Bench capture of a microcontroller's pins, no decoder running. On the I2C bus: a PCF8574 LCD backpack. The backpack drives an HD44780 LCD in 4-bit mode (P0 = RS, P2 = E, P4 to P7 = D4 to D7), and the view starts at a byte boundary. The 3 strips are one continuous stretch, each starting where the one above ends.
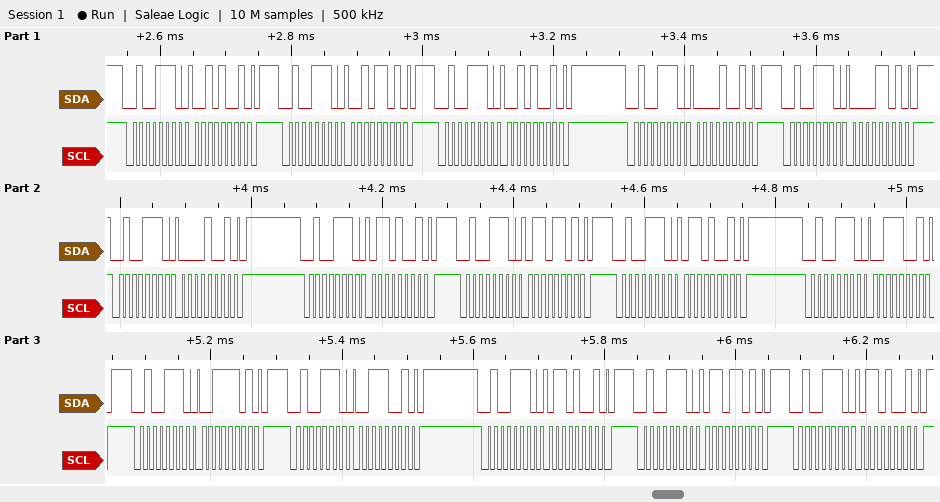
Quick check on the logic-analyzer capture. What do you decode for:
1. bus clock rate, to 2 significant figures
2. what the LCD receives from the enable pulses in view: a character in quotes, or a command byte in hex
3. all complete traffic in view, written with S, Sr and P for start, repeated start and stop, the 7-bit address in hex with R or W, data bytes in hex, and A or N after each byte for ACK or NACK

100 kHz
' ' 'c'
S 27W A 29 A P S 27W A 2D A P S 27W A 29 A P S 27W A 09 A P S 27W A 0D A P S 27W A 09 A P S 27W A 69 A P S 27W A 6D A P S 27W A 69 A P S 27W A 39 A P S 27W A 3D A P S 27W A 39 A P S 27W A 69 A P S 27W A 6D A P S 27W A 69 A P
